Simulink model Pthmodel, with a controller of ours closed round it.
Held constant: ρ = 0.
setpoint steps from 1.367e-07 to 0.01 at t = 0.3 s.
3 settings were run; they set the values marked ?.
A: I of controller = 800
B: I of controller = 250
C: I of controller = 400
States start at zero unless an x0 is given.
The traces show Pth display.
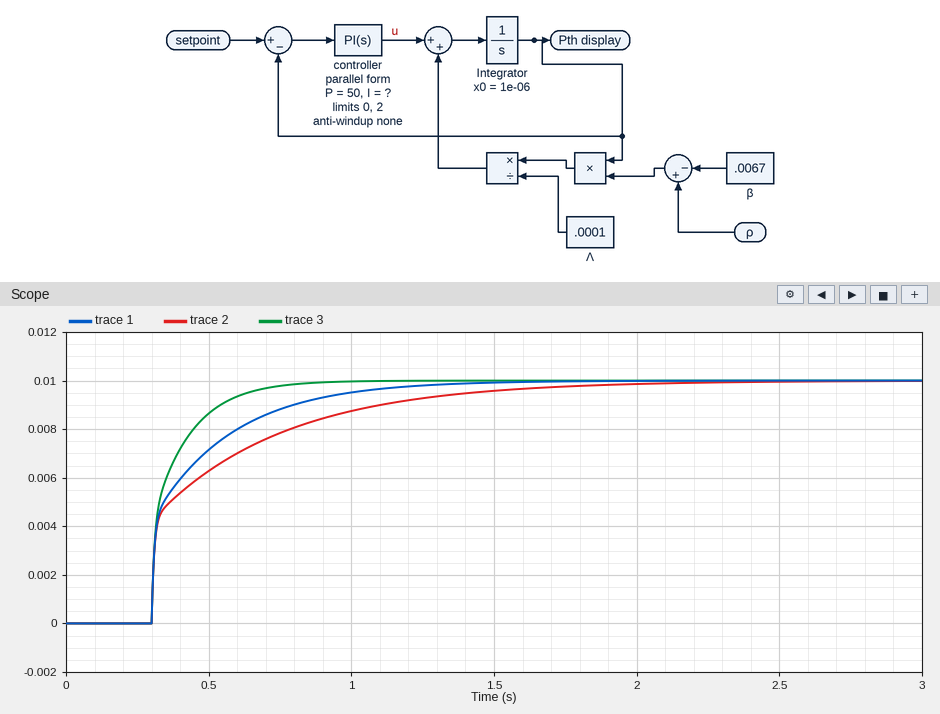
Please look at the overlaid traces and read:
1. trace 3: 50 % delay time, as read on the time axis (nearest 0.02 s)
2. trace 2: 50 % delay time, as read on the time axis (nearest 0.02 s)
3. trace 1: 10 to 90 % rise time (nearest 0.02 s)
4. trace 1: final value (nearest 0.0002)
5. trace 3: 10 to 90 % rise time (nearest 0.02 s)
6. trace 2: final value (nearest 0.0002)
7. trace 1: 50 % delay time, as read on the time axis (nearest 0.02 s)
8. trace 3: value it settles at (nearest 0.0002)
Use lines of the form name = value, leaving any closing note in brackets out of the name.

trace 3: 50 % delay time, as read on the time axis = 0.32 s
trace 2: 50 % delay time, as read on the time axis = 0.36 s
trace 1: 10 to 90 % rise time = 0.50 s
trace 1: final value = 0.0100
trace 3: 10 to 90 % rise time = 0.24 s
trace 2: final value = 0.0100
trace 1: 50 % delay time, as read on the time axis = 0.34 s
trace 3: value it settles at = 0.0100
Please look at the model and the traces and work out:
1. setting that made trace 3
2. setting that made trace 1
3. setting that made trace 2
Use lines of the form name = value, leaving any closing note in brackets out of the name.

setting that made trace 3 = A
setting that made trace 1 = C
setting that made trace 2 = B
